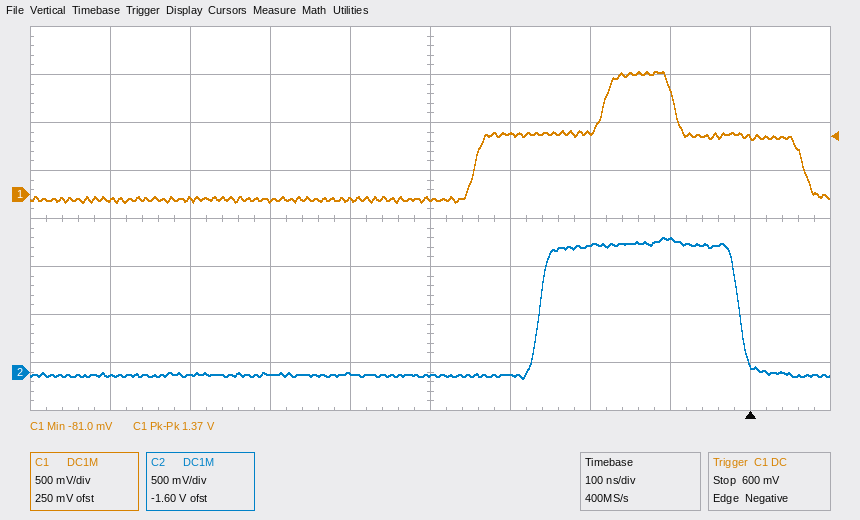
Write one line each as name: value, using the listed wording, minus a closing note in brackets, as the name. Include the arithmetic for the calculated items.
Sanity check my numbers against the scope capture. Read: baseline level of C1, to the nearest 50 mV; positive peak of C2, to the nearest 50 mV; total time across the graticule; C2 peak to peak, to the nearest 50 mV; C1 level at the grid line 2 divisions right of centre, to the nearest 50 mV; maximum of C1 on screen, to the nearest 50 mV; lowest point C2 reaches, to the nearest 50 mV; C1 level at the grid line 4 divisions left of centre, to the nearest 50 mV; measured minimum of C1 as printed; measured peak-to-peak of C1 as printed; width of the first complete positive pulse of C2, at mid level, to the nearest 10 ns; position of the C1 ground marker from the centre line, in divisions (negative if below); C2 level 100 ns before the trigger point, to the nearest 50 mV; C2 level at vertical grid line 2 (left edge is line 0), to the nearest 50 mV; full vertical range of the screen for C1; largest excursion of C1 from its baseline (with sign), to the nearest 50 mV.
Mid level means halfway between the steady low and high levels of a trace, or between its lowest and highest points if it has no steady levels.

baseline level of C1, to the nearest 50 mV: -50 mV
positive peak of C2, to the nearest 50 mV: 1.40 V
total time across the graticule: 1 µs
C2 peak to peak, to the nearest 50 mV: 1.40 V − (-50 mV) = 1.45 V
C1 level at the grid line 2 divisions right of centre, to the nearest 50 mV: 650 mV
maximum of C1 on screen, to the nearest 50 mV: 1.30 V
lowest point C2 reaches, to the nearest 50 mV: -50 mV
C1 level at the grid line 4 divisions left of centre, to the nearest 50 mV: -50 mV
measured minimum of C1 as printed: -81.0 mV
measured peak-to-peak of C1 as printed: 1.37 V
width of the first complete positive pulse of C2, at mid level, to the nearest 10 ns: 250 ns
position of the C1 ground marker from the centre line, in divisions: +0.5 div
C2 level 100 ns before the trigger point, to the nearest 50 mV: 1.40 V
C2 level at vertical grid line 2 (left edge is line 0), to the nearest 50 mV: -50 mV
full vertical range of the screen for C1: 4 V
largest excursion of C1 from its baseline (with sign), to the nearest 50 mV: 1.30 V − (-50 mV) = +1.35 V
